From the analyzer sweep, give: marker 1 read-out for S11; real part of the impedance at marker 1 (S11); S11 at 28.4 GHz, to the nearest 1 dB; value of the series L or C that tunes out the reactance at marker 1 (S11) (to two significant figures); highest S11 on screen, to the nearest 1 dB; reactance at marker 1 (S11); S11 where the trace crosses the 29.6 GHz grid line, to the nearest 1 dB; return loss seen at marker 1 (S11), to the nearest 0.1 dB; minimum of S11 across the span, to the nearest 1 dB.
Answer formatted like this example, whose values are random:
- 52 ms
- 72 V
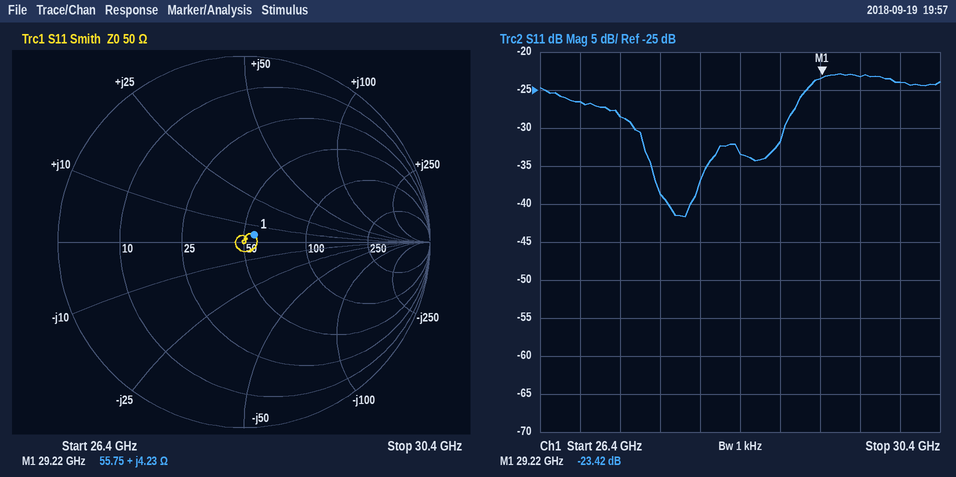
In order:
- -23.42 dB
- 55.75 Ω
- -33 dB
- 1.3 pF
- -23 dB
- +4.23 Ω
- -23 dB
- 23.4 dB
- -42 dB
